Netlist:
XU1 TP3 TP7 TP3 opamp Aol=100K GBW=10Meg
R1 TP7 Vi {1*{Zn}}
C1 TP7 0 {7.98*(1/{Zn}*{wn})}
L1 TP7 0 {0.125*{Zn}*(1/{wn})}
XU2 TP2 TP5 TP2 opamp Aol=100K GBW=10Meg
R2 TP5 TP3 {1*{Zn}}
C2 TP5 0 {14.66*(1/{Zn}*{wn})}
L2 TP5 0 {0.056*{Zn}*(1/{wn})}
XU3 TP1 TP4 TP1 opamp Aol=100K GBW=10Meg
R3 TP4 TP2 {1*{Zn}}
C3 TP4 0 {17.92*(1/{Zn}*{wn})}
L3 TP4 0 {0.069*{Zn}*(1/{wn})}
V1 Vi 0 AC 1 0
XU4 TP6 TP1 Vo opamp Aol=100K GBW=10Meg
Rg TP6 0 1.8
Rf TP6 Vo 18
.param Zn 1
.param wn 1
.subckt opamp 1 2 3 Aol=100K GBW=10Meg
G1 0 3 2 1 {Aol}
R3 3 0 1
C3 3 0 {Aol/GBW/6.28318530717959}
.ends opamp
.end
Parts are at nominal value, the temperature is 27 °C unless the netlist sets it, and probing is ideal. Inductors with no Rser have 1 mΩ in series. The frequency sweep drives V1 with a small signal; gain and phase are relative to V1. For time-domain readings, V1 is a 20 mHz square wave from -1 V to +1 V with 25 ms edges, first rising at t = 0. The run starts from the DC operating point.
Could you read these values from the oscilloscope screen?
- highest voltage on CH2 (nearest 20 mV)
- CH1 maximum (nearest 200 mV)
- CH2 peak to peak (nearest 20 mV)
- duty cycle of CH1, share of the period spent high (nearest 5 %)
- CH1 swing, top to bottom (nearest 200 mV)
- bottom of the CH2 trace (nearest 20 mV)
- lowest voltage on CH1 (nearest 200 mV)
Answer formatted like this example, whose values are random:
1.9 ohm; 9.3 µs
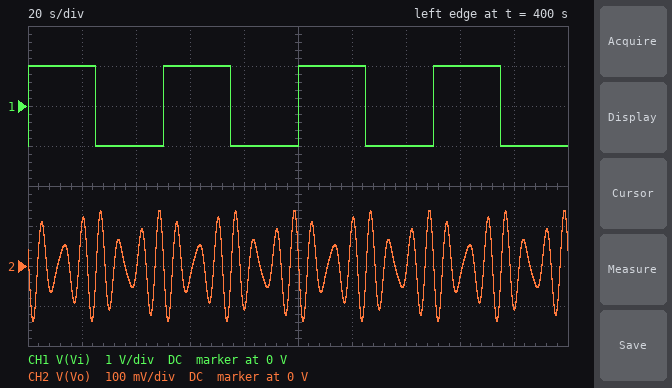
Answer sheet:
140 mV; 1.0 V; 280 mV; 50 %; 2.0 V; -140 mV; -1.0 V
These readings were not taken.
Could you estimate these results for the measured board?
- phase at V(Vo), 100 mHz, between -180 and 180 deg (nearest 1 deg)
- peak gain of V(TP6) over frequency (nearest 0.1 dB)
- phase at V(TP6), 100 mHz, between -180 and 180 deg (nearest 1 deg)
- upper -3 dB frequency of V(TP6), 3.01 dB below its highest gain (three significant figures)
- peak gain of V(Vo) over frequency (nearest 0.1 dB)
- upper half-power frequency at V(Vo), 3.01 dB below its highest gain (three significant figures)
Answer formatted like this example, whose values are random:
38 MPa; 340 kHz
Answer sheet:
-111 deg; -22.5 dB; -111 deg; 178 mHz; -1.7 dB; 178 mHz
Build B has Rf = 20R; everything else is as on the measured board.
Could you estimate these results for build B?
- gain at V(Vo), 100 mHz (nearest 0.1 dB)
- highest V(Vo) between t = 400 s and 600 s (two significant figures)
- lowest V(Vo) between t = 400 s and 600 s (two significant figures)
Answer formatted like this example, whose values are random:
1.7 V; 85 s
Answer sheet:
-43.4 dB; 150 mV; -150 mV
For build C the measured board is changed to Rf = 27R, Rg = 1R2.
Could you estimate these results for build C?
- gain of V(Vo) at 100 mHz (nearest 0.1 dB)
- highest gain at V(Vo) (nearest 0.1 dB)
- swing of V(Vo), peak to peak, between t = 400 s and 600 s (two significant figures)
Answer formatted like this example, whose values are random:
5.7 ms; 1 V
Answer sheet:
-37.6 dB; 4.9 dB; 590 mV
